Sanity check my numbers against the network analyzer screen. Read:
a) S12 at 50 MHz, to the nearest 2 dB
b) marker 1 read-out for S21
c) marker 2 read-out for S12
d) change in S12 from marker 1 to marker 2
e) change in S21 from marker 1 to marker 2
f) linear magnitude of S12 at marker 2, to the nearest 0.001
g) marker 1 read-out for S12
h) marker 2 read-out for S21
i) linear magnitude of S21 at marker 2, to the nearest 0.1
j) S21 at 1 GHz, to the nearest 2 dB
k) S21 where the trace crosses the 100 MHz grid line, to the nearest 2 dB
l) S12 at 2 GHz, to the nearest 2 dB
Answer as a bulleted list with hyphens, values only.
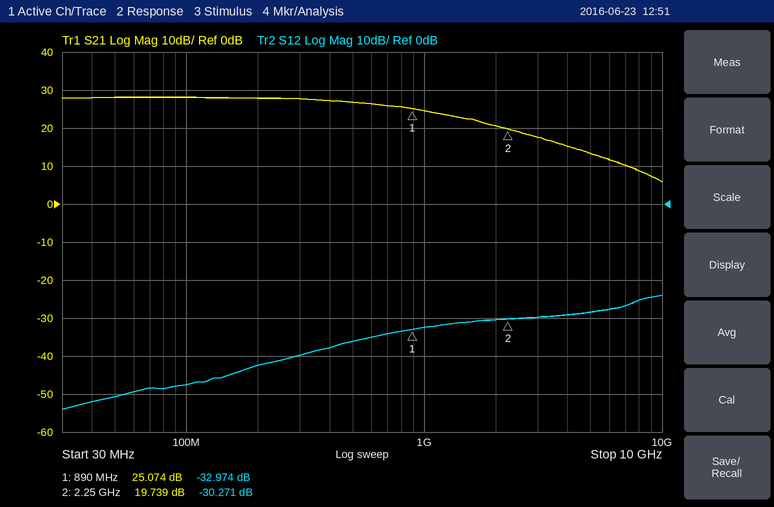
- -50 dB
- 25.074 dB
- -30.271 dB
- 2.703 dB
- -5.335 dB
- 0.031
- -32.974 dB
- 19.739 dB
- 9.7
- 24 dB
- 28 dB
- -30 dB
